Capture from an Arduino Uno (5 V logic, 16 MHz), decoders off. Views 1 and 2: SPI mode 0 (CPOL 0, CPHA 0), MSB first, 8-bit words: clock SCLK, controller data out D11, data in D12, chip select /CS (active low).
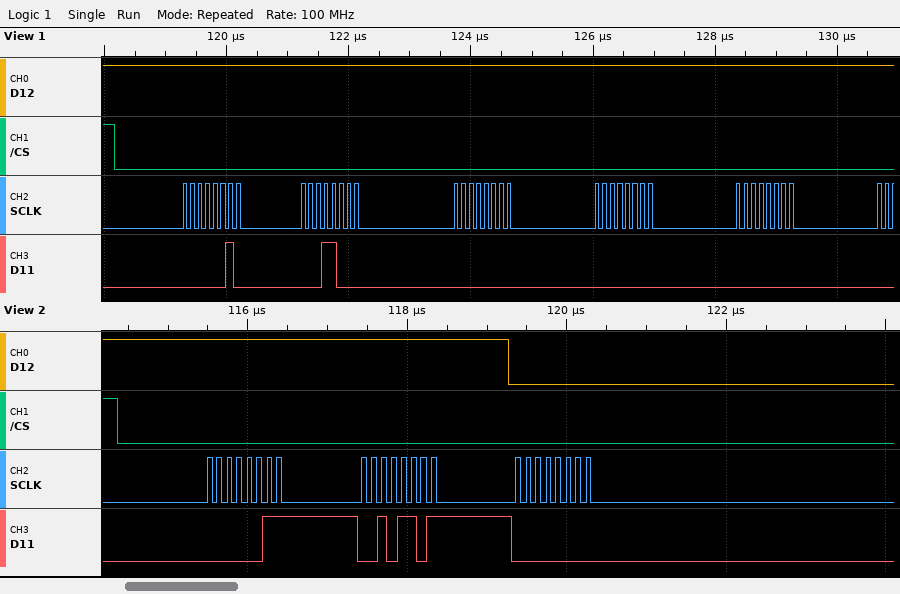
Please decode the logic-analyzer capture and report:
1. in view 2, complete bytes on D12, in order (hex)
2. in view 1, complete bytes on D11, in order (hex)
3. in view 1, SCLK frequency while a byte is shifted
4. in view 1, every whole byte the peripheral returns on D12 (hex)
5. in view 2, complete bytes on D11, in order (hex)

0xFF 0xFF 0x00
02 18 00 00 00
8 MHz
FF FF FF FF FF
0x03 0x2D 0x00
